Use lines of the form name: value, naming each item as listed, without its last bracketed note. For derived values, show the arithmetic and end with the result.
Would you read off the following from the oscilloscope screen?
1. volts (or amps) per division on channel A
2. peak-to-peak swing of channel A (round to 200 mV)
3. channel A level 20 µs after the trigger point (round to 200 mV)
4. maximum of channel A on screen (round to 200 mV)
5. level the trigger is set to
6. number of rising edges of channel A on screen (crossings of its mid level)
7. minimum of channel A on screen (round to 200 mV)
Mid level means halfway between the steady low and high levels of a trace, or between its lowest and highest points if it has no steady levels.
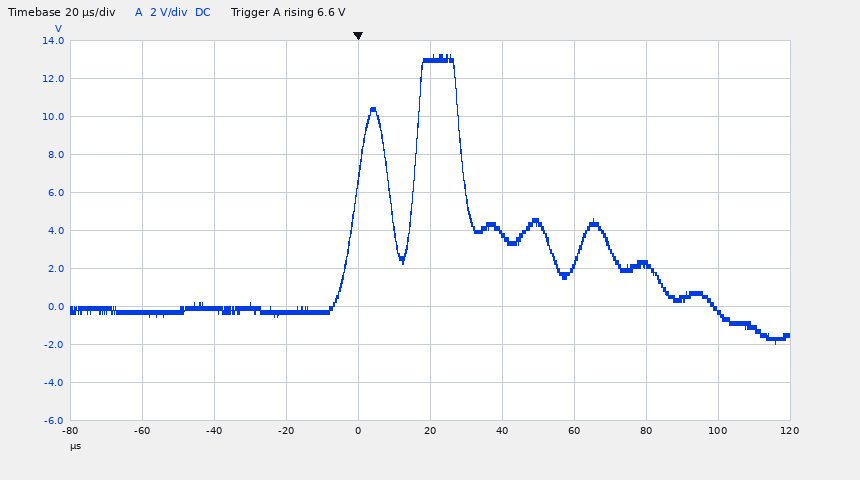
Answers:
volts (or amps) per division on channel A: 2 V
peak-to-peak swing of channel A: 13.2 V − (-2.0 V) = 15.2 V
channel A level 20 µs after the trigger point: 13.0 V
maximum of channel A on screen: 13.2 V
level the trigger is set to: 6.6 V
number of rising edges of channel A on screen: 2
minimum of channel A on screen: -2.0 V
